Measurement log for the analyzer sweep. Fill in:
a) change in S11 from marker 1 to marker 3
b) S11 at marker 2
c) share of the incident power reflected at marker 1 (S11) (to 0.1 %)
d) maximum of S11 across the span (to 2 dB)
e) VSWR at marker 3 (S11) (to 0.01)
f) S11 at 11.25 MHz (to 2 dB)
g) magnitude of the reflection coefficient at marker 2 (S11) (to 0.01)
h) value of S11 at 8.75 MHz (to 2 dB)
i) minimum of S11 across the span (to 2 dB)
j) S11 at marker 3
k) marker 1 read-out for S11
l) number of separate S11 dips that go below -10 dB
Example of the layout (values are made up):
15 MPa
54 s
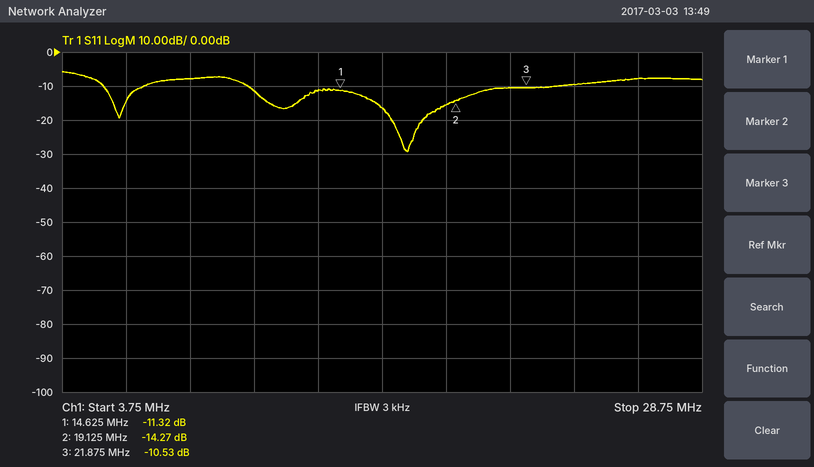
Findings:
0.79 dB
-14.27 dB
7.4 %
-6 dB
1.85
-12 dB
0.19
-8 dB
-30 dB
-10.53 dB
-11.32 dB
3
